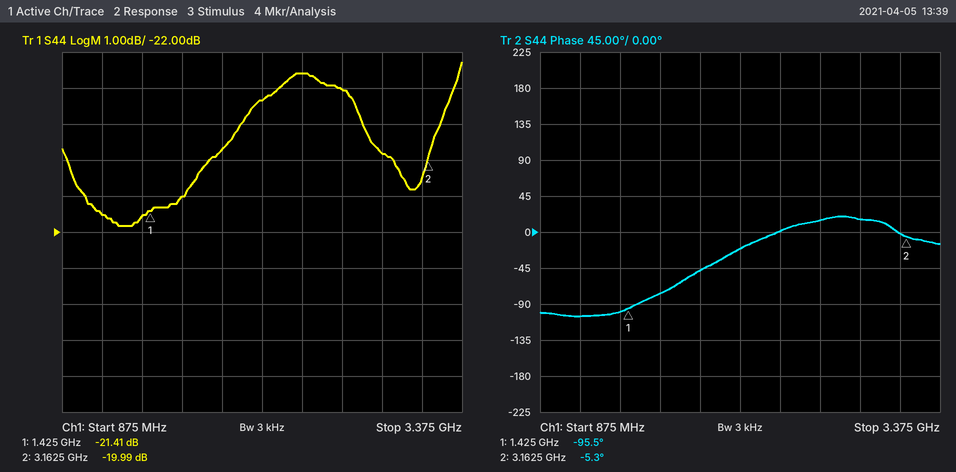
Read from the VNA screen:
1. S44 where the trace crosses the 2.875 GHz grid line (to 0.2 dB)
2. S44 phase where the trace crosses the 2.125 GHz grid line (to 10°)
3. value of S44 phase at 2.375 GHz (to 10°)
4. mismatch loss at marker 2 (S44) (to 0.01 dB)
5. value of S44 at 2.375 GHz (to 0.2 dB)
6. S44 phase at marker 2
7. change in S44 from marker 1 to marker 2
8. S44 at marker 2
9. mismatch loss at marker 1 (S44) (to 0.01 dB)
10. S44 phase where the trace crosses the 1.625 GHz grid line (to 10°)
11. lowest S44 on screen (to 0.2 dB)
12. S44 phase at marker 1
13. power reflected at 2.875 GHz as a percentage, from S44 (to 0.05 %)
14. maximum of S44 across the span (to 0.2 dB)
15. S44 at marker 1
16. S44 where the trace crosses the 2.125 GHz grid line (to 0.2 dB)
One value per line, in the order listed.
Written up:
-19.8 dB
-20°
0°
0.04 dB
-17.6 dB
-5.3°
1.42 dB
-19.99 dB
0.03 dB
-80°
-21.8 dB
-95.5°
1.05 %
-17.2 dB
-21.41 dB
-18.4 dB
